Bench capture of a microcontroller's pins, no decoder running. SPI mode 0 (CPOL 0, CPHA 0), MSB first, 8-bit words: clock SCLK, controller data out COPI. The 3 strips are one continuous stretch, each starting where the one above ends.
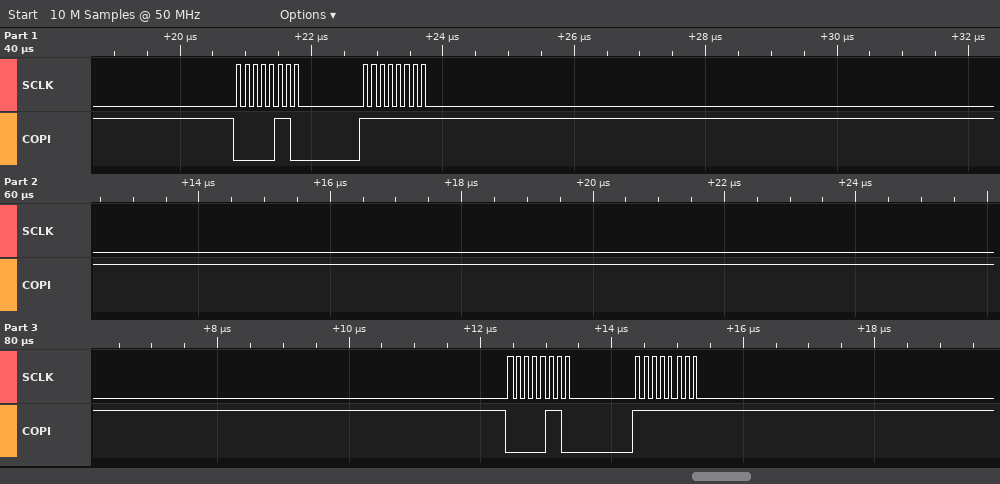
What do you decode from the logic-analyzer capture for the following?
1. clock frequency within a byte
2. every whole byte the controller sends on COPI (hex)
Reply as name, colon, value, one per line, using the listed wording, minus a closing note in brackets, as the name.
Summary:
clock frequency within a byte: 8 MHz
every whole byte the controller sends on COPI: 06 FF 06 FF
